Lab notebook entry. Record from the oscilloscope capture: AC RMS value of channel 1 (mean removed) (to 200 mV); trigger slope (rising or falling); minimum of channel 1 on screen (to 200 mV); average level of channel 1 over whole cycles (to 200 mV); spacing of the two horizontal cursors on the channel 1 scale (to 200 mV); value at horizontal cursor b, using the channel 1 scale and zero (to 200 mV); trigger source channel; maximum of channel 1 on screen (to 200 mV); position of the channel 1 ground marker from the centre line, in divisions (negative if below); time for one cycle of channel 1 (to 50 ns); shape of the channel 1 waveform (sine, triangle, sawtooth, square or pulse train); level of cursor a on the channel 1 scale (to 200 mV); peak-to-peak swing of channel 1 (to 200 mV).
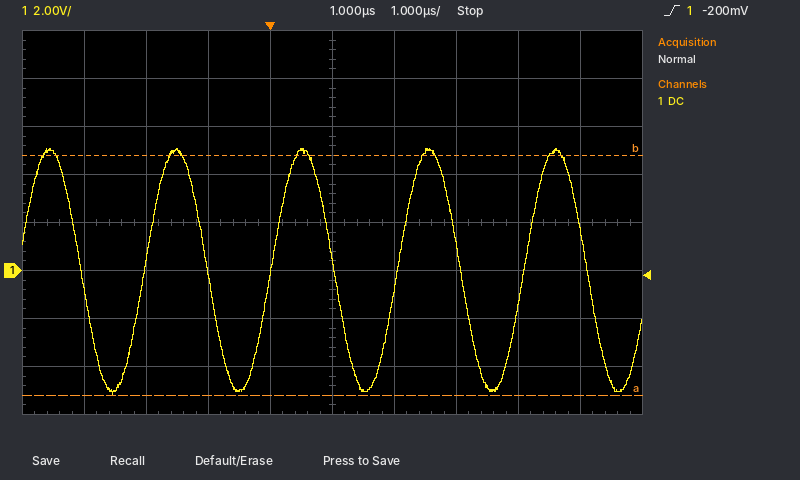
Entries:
3.6 V
rising
-5.2 V
0.0 V
10.0 V
4.8 V
channel 1
5.0 V
-1.0 div
2.05 µs
sine
-5.2 V
10.2 V
